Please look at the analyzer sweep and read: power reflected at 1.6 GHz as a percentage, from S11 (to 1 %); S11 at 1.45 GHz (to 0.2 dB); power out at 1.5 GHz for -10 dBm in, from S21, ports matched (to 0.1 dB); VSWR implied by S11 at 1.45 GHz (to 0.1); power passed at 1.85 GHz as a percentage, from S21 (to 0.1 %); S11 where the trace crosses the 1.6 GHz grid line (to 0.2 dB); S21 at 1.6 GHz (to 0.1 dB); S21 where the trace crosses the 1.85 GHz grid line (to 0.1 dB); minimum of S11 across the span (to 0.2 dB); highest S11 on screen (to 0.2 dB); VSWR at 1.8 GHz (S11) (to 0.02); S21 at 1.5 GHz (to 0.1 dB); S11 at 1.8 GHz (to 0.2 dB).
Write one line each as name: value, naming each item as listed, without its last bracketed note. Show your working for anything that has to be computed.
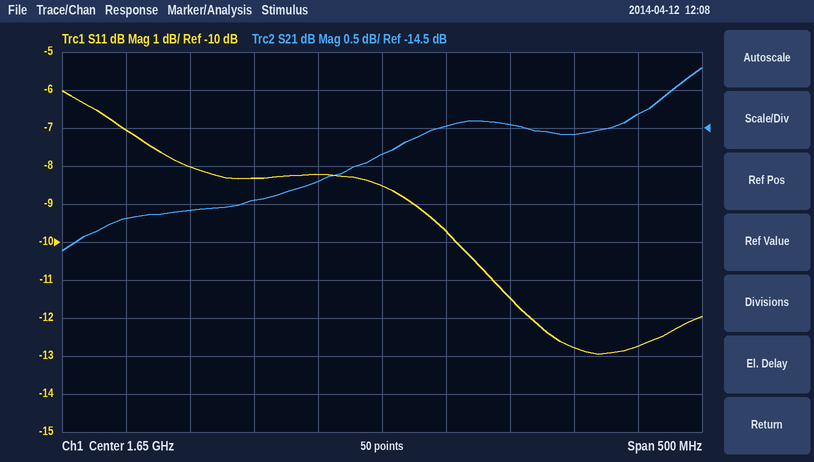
power reflected at 1.6 GHz as a percentage, from S11: 10^(-8.2/10) ≈ 15 %
S11 at 1.45 GHz: -7.0 dB
power out at 1.5 GHz for -10 dBm in, from S21, ports matched: -10 dBm + (-15.6 dB) = -25.6 dBm
VSWR implied by S11 at 1.45 GHz: |Γ| = 10^(-7/20) = 0.4467; VSWR = (1 + 0.4467)/(1 − 0.4467) ≈ 2.6
power passed at 1.85 GHz as a percentage, from S21: 10^(-14.3/10) ≈ 3.7 %
S11 where the trace crosses the 1.6 GHz grid line: -8.2 dB
S21 at 1.6 GHz: -15.2 dB
S21 where the trace crosses the 1.85 GHz grid line: -14.3 dB
minimum of S11 across the span: -13.0 dB
highest S11 on screen: -6.0 dB
VSWR at 1.8 GHz (S11): |Γ| = 10^(-12.8/20) = 0.2291; VSWR = (1 + 0.2291)/(1 − 0.2291) ≈ 1.59, so 1.60 to the nearest 0.02
S21 at 1.5 GHz: -15.6 dB
S11 at 1.8 GHz: -12.8 dB
